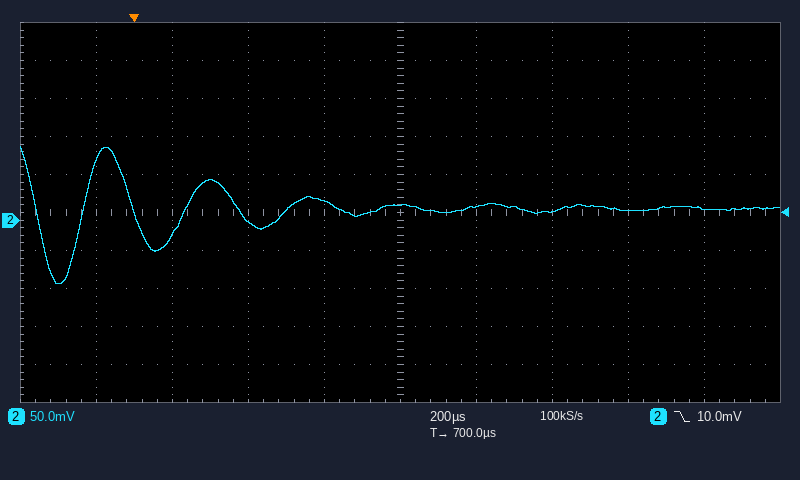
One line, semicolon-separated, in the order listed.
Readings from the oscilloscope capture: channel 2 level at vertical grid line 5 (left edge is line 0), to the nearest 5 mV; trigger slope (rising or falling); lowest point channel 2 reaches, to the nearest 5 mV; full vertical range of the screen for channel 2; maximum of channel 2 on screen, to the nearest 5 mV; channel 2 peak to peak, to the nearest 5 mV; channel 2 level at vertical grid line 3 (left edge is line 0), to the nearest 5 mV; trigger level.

20 mV; falling; -85 mV; 500 mV; 95 mV; 180 mV; 0 mV; 10.0 mV
